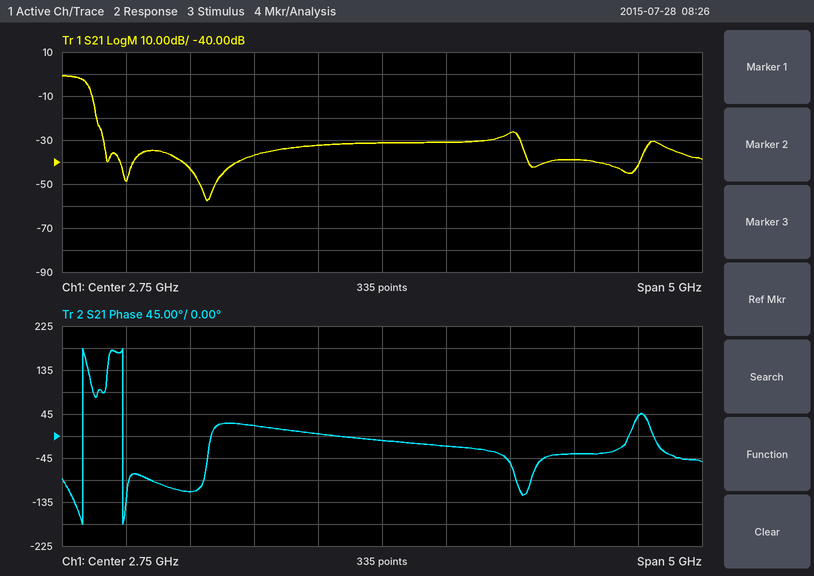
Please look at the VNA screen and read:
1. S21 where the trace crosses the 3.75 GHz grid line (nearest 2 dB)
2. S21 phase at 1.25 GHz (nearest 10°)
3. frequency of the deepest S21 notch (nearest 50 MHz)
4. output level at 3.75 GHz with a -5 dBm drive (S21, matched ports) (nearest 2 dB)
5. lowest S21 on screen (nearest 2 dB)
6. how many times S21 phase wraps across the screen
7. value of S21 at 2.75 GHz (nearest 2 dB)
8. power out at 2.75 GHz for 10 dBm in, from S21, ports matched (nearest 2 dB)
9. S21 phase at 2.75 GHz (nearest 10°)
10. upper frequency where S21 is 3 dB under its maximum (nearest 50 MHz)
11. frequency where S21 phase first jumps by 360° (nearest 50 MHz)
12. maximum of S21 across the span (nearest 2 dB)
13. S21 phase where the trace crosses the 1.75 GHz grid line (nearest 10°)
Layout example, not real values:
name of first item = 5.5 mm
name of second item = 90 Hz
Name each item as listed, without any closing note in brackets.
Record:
S21 where the trace crosses the 3.75 GHz grid line = -26 dB
S21 phase at 1.25 GHz = -110°
frequency of the deepest S21 notch = 1.40 GHz
output level at 3.75 GHz with a -5 dBm drive (S21, matched ports) = -32 dBm
lowest S21 on screen = -58 dB
how many times S21 phase wraps across the screen = 2
value of S21 at 2.75 GHz = -32 dB
power out at 2.75 GHz for 10 dBm in, from S21, ports matched = -22 dBm
S21 phase at 2.75 GHz = -10°
upper frequency where S21 is 3 dB under its maximum = 450 MHz
frequency where S21 phase first jumps by 360° = 400 MHz
maximum of S21 across the span = 0 dB
S21 phase where the trace crosses the 1.75 GHz grid line = 20°
